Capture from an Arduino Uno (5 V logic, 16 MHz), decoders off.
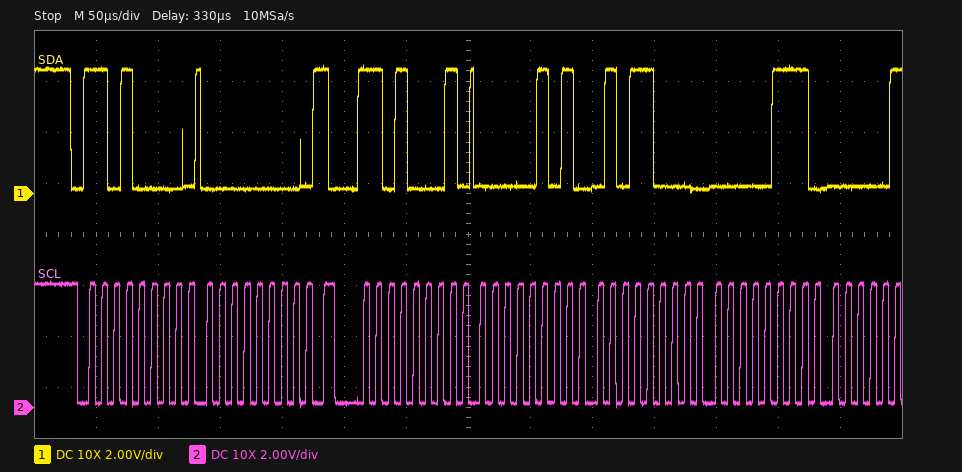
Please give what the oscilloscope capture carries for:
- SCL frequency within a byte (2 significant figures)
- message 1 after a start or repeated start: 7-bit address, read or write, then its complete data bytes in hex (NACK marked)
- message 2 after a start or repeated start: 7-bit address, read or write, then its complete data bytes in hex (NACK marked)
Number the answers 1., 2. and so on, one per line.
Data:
1. 100 kHz
2. 0x68 write: 00
3. 0x68 read: 05 58 07
